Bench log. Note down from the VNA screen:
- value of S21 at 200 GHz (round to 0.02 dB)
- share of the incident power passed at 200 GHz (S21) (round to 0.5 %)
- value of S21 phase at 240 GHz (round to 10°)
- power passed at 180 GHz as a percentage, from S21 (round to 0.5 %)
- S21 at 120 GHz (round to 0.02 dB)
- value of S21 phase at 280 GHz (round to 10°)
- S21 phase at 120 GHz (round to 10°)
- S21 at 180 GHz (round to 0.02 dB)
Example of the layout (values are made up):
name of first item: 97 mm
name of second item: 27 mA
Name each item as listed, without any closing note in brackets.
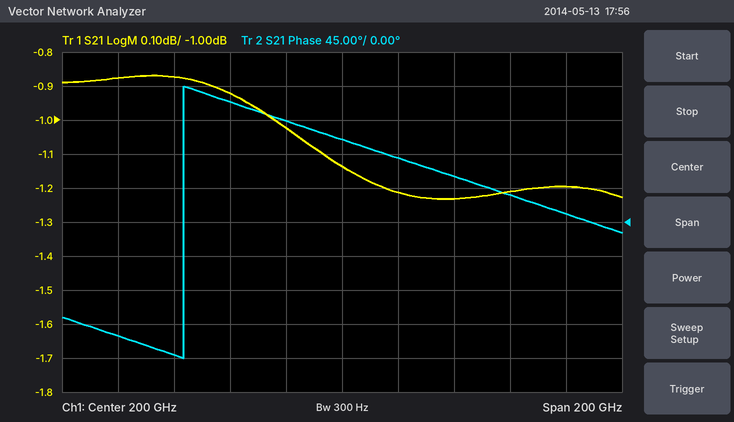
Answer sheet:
value of S21 at 200 GHz: -1.14 dB
share of the incident power passed at 200 GHz (S21): 77.0 %
value of S21 phase at 240 GHz: 60°
power passed at 180 GHz as a percentage, from S21: 79.0 %
S21 at 120 GHz: -0.88 dB
value of S21 phase at 280 GHz: 10°
S21 phase at 120 GHz: -150°
S21 at 180 GHz: -1.02 dB
